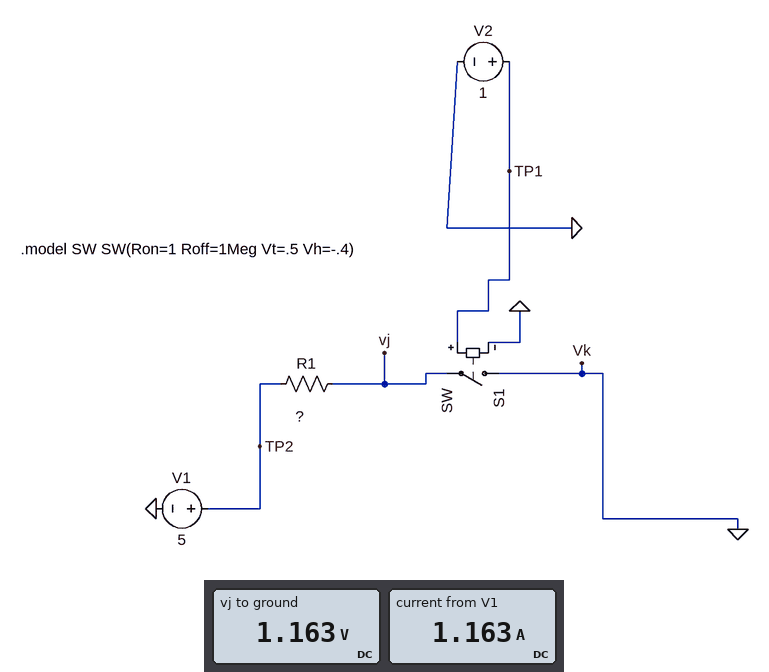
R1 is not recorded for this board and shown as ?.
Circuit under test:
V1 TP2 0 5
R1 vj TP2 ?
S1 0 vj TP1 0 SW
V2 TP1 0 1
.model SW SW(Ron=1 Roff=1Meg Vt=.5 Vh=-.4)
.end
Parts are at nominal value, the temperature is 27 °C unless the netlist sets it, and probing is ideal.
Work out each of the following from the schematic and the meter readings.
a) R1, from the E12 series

3.3 Ω
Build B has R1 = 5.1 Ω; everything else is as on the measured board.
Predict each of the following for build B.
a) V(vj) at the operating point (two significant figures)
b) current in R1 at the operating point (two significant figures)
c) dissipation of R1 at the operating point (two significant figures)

820 mV
820 mA
3.4 W
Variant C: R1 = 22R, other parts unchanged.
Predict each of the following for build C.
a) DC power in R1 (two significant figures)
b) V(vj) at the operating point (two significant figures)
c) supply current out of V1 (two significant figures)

1.0 W
220 mV
220 mA
